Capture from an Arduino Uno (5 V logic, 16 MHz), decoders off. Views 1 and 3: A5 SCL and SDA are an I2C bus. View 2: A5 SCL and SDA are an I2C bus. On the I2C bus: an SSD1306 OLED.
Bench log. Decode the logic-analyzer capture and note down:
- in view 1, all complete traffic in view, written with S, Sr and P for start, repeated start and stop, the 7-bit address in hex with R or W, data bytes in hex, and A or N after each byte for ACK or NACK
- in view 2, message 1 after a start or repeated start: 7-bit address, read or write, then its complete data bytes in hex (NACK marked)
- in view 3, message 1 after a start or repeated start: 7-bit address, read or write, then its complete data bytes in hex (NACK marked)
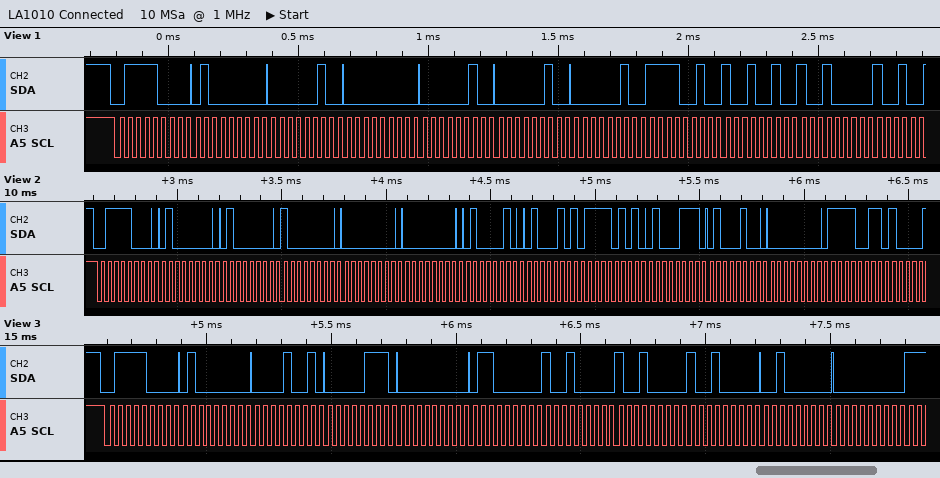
S 3CW A 40 A 02 A 00 A 02 A 02 A 02 A F2 A 92 A 90 A
0x3C write: 40 40 80 00 00 42 45 F5 47 44 00 F3
0x3C write: 40 09 07 00 60 90 90 90 20 00
